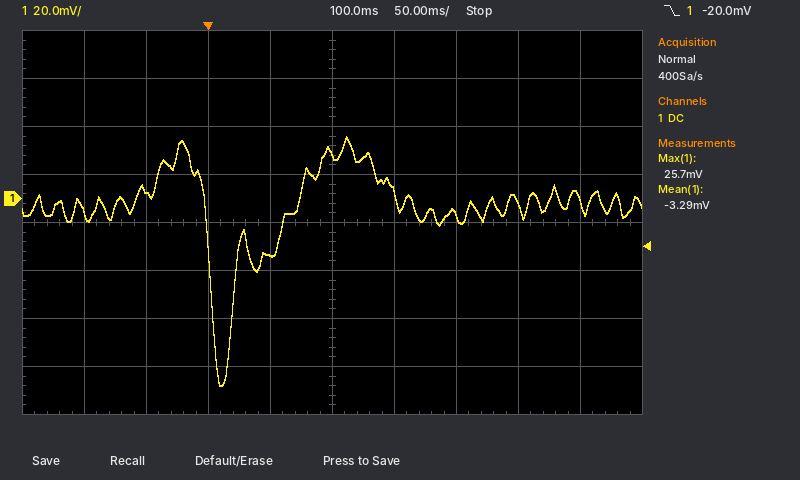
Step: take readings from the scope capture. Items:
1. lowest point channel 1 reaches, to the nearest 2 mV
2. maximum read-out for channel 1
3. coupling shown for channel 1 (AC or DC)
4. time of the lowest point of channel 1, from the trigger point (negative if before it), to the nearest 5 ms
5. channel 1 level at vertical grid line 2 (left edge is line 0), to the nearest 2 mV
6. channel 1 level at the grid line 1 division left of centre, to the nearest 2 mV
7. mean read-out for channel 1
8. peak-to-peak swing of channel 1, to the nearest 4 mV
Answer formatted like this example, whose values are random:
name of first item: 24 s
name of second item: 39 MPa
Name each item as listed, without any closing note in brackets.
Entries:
lowest point channel 1 reaches, to the nearest 2 mV: -78 mV
maximum read-out for channel 1: 25.7 mV
coupling shown for channel 1: DC
time of the lowest point of channel 1, from the trigger point (negative if before it), to the nearest 5 ms: +10 ms
channel 1 level at vertical grid line 2 (left edge is line 0), to the nearest 2 mV: 4 mV
channel 1 level at the grid line 1 division left of centre, to the nearest 2 mV: -24 mV
mean read-out for channel 1: -3.29 mV
peak-to-peak swing of channel 1, to the nearest 4 mV: 104 mV
